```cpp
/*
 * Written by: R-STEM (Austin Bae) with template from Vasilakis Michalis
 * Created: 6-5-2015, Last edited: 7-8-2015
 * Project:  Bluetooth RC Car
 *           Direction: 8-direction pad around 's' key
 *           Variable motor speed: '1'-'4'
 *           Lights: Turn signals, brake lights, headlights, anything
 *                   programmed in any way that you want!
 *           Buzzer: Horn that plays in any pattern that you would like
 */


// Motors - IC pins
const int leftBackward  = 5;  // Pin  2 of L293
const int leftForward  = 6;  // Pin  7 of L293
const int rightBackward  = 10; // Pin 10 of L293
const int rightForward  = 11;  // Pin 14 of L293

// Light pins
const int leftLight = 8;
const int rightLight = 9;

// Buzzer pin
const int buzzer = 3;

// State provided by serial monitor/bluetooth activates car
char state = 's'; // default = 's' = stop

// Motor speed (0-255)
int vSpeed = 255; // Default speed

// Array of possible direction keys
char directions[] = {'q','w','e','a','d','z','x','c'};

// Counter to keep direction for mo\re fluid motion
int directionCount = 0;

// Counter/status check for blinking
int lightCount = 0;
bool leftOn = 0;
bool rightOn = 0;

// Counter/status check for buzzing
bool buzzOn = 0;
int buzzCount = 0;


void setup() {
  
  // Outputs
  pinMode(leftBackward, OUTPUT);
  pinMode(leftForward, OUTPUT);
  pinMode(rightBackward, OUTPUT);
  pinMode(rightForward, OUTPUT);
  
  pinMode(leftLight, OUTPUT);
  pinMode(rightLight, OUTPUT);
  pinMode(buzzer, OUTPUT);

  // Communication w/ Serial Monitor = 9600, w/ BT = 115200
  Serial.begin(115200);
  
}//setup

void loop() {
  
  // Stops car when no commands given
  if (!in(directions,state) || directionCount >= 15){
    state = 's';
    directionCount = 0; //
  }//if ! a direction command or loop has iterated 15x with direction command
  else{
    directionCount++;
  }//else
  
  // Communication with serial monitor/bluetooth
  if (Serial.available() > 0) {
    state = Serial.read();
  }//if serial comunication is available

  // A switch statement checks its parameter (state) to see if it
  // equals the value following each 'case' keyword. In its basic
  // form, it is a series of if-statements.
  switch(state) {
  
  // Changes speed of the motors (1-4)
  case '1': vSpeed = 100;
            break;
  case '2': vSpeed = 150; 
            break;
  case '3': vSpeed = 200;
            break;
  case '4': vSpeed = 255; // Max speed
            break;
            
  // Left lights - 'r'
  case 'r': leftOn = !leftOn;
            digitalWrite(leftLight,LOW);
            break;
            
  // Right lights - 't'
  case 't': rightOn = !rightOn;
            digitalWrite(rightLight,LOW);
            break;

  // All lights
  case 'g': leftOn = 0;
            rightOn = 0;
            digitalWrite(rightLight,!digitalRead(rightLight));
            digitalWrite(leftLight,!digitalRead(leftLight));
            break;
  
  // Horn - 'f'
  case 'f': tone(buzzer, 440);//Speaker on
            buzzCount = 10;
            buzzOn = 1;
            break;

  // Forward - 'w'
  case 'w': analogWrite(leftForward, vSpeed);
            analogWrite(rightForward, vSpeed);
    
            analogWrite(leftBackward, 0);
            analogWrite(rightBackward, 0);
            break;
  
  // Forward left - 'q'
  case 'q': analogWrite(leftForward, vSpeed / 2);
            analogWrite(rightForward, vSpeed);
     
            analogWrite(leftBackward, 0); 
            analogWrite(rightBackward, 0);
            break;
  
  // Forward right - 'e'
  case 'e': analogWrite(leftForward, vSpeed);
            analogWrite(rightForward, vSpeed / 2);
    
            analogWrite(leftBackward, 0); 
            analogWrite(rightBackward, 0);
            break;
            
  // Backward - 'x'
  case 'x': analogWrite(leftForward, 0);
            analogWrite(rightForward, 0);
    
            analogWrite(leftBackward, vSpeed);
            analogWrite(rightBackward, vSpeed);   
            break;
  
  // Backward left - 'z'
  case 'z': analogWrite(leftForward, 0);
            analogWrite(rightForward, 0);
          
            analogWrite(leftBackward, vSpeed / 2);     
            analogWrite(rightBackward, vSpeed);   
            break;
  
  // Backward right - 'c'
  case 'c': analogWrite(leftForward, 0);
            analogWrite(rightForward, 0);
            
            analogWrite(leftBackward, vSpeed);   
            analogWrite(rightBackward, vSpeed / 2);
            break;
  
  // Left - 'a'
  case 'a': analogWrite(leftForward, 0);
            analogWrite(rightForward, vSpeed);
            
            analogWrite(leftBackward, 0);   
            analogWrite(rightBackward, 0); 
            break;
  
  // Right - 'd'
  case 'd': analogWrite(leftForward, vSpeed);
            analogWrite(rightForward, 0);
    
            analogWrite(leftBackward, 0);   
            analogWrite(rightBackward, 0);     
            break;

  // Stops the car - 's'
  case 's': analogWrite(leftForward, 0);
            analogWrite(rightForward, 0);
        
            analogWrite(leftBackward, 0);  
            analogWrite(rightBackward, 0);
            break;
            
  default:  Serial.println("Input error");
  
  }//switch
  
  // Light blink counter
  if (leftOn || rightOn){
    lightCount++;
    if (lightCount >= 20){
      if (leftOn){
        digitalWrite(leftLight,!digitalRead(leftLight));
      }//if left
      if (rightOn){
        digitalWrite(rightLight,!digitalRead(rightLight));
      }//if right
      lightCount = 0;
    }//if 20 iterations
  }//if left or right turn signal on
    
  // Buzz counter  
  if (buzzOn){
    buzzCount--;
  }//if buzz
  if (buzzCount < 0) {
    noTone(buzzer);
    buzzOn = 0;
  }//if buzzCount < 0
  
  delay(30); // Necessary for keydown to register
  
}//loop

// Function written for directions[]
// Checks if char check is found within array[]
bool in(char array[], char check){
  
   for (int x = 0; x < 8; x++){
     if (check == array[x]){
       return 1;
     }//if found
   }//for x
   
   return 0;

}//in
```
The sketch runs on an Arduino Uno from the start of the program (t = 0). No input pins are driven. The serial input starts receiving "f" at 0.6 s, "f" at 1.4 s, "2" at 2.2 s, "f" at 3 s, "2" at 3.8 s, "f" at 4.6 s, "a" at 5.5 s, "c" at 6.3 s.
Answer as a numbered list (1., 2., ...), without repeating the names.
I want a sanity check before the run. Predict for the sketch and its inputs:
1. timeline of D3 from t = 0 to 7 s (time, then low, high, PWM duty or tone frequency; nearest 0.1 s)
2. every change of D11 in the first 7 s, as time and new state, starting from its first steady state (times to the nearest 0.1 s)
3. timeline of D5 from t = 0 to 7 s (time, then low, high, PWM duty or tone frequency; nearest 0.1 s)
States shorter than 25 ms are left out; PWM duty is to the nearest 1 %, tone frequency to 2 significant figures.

1. 0 s low; 0.6 s tone 440 Hz; 0.9 s low; 1.4 s tone 440 Hz; 1.7 s low; 3 s tone 440 Hz; 3.3 s low; 4.6 s tone 440 Hz; 4.9 s low
2. 0 s low; 5.5 s PWM 59 %; 6 s low
3. 0 s low; 6.3 s PWM 59 %; 6.8 s low
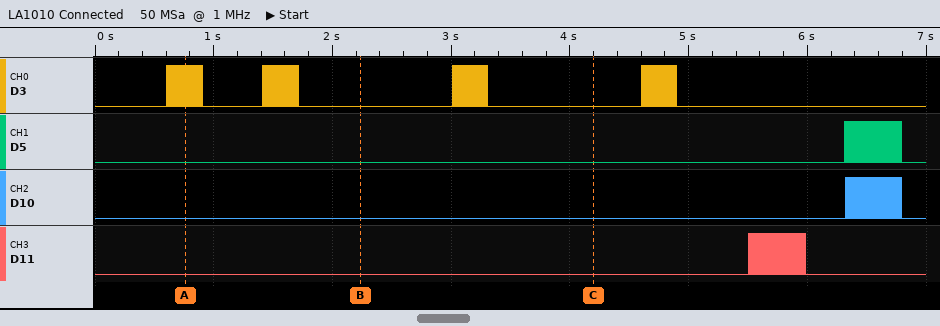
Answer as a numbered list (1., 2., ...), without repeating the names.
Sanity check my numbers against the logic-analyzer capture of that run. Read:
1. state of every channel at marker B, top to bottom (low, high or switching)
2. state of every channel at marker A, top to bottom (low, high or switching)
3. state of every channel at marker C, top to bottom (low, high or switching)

1. D3 low, D5 low, D10 low, D11 low
2. D3 switching, D5 low, D10 low, D11 low
3. D3 low, D5 low, D10 low, D11 low
